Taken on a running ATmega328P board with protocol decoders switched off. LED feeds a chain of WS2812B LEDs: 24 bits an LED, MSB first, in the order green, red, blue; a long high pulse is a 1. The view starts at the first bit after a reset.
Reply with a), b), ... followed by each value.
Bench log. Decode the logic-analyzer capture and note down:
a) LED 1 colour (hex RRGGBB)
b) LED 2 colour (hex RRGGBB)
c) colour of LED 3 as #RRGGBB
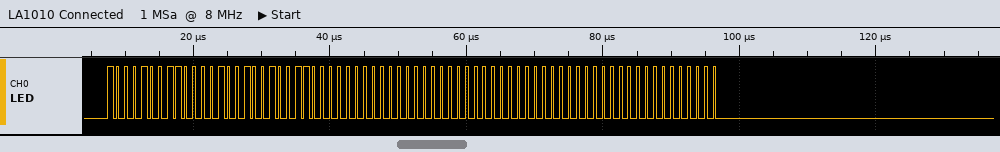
a) #848993
b) #000000
c) #000000
